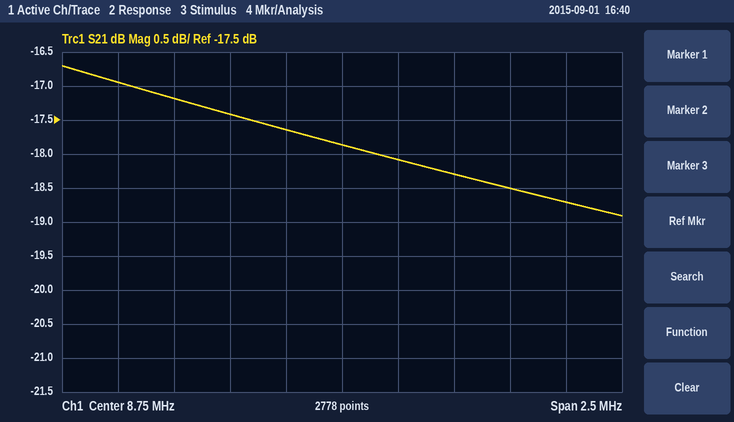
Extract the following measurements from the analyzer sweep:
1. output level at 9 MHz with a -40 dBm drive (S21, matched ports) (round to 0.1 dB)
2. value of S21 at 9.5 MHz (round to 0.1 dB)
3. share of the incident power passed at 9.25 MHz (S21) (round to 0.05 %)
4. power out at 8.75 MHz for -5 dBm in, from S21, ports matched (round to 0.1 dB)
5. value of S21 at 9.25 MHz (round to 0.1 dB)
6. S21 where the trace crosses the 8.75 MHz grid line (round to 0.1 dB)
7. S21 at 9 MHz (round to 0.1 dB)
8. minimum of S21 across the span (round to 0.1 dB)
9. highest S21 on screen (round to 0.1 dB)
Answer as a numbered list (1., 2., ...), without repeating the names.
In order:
1. -58.1 dBm
2. -18.5 dB
3. 1.50 %
4. -22.9 dBm
5. -18.3 dB
6. -17.9 dB
7. -18.1 dB
8. -18.9 dB
9. -16.7 dB
